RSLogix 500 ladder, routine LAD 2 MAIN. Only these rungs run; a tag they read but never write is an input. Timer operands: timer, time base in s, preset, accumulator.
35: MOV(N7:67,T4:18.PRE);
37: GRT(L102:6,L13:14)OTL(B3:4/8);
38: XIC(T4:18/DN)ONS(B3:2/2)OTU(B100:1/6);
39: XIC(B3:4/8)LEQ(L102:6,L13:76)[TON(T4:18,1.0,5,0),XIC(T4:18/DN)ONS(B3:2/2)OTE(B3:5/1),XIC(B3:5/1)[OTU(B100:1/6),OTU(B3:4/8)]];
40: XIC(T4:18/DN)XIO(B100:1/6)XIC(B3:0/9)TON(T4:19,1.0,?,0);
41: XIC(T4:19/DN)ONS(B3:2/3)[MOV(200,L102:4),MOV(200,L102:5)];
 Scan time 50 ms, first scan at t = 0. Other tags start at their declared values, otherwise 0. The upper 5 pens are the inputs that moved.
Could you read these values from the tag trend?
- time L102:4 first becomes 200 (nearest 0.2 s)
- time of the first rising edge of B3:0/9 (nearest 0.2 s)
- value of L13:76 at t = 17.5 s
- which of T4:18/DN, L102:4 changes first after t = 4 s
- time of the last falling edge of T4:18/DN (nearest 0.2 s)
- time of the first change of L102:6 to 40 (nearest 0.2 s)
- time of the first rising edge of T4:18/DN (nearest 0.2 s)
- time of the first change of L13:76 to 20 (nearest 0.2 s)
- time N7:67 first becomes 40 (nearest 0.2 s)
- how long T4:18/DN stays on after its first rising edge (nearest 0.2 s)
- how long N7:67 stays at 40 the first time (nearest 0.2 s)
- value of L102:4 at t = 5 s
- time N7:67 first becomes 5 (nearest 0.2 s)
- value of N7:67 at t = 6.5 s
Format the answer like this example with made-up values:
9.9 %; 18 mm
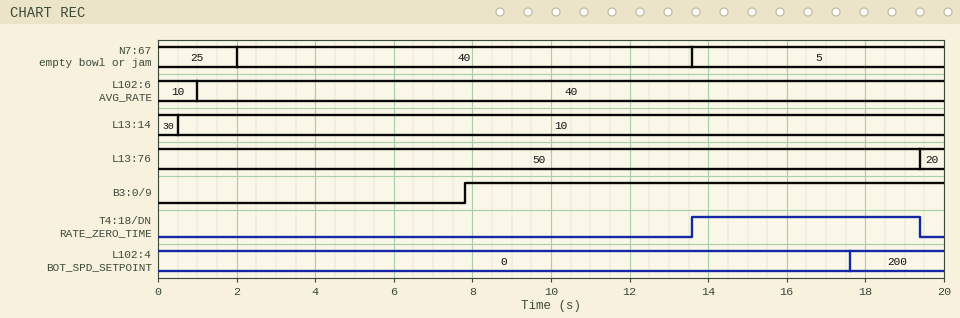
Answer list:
17.6 s; 7.8 s; 50; T4:18/DN; 19.4 s; 1.0 s; 13.6 s; 19.4 s; 2.0 s; 5.8 s; 11.6 s; 0; 13.6 s; 40
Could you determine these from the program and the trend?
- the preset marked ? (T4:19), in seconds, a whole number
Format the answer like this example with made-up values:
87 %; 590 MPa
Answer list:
4 s
